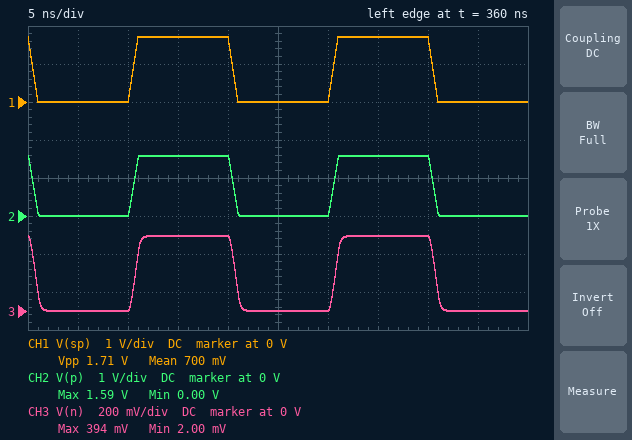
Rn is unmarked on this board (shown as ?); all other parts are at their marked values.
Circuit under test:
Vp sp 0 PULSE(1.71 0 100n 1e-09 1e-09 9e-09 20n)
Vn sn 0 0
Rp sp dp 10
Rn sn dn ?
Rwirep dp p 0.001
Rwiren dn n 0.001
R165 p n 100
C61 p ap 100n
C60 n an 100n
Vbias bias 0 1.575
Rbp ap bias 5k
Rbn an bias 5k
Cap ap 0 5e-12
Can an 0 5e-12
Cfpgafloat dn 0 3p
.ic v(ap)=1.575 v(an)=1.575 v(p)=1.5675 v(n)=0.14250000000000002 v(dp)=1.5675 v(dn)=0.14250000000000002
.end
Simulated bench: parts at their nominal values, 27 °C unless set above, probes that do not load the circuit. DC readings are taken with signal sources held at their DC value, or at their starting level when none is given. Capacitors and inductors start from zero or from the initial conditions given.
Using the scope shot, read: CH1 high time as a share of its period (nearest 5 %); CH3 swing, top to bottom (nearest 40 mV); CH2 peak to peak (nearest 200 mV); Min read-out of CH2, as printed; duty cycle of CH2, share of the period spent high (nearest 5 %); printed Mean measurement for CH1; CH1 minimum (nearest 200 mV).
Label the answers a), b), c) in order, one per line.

a) 50 %
b) 400 mV
c) 1.6 V
d) 0.00 V
e) 50 %
f) 700 mV
g) 0 V
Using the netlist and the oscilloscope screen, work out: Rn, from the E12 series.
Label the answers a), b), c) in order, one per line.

a) 33 Ω
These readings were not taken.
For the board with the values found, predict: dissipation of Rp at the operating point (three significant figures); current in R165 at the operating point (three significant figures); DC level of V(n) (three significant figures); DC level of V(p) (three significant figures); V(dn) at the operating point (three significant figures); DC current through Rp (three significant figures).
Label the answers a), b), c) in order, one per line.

a) 1.43 mW
b) 12.0 mA
c) 395 mV
d) 1.59 V
e) 395 mV
f) 12.0 mA
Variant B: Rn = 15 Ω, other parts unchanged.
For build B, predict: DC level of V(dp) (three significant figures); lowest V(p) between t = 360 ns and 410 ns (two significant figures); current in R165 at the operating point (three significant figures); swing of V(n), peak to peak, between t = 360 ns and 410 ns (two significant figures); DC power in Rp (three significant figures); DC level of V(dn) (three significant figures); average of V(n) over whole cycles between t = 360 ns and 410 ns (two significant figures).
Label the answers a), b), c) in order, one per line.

a) 1.57 V
b) 2.9 mV
c) 13.7 mA
d) 200 mV
e) 1.87 mW
f) 205 mV
g) 100 mV
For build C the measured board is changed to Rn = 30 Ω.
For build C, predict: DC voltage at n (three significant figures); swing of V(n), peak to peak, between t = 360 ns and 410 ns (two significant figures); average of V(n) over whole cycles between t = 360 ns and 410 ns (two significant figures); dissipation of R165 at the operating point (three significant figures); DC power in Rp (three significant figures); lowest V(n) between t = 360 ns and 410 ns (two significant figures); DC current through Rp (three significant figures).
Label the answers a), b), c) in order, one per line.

a) 366 mV
b) 360 mV
c) 180 mV
d) 14.9 mW
e) 1.49 mW
f) 1.3 mV
g) 12.2 mA
